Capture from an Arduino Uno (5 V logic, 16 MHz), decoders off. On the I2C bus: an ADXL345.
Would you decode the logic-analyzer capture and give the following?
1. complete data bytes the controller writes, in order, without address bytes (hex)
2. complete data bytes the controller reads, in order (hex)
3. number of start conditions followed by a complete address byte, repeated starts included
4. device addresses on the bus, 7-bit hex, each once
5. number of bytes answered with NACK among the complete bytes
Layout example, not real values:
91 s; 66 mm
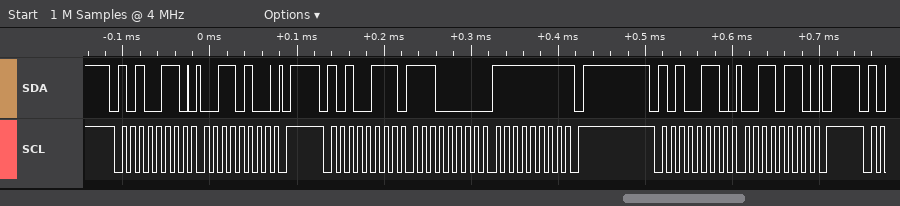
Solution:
34 36; E0 FF; 3; 0x53; 1
